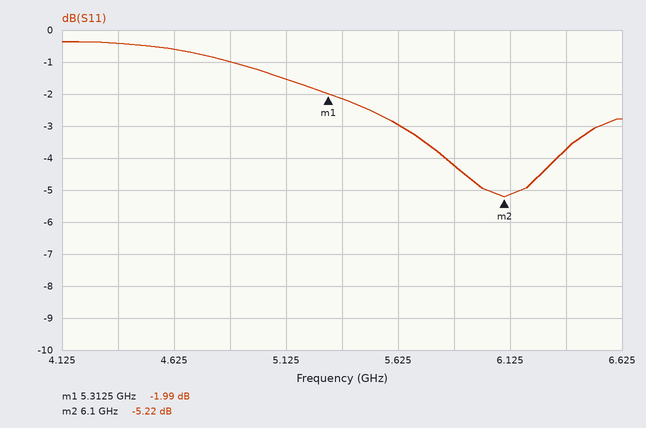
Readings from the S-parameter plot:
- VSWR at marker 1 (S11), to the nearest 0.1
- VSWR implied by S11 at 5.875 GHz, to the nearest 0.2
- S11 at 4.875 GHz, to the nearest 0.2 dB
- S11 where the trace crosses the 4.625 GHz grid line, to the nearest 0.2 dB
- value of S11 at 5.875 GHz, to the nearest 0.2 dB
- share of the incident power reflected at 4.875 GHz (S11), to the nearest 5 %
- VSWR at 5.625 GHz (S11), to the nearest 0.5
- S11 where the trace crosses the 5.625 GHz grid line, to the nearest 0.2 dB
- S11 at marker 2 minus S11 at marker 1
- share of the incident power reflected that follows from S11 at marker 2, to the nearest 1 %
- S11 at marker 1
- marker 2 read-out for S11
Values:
8.8
4.2
-1.0 dB
-0.6 dB
-4.2 dB
80 %
6.0
-3.0 dB
-3.23 dB
30 %
-1.99 dB
-5.22 dB
